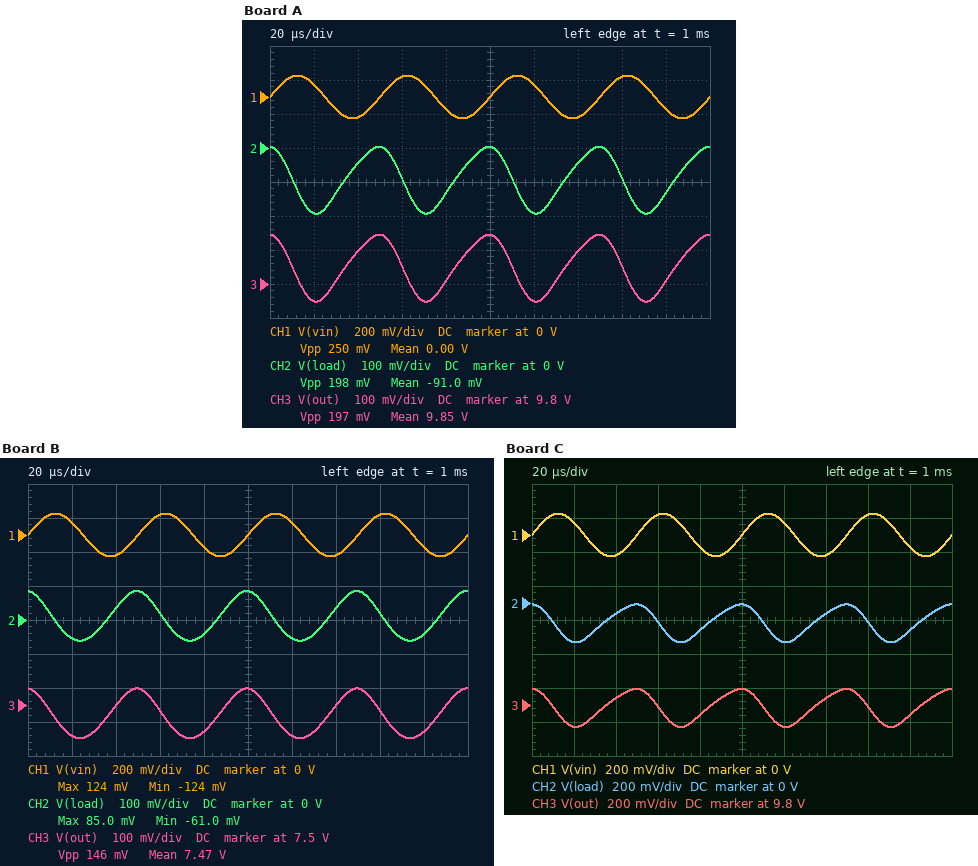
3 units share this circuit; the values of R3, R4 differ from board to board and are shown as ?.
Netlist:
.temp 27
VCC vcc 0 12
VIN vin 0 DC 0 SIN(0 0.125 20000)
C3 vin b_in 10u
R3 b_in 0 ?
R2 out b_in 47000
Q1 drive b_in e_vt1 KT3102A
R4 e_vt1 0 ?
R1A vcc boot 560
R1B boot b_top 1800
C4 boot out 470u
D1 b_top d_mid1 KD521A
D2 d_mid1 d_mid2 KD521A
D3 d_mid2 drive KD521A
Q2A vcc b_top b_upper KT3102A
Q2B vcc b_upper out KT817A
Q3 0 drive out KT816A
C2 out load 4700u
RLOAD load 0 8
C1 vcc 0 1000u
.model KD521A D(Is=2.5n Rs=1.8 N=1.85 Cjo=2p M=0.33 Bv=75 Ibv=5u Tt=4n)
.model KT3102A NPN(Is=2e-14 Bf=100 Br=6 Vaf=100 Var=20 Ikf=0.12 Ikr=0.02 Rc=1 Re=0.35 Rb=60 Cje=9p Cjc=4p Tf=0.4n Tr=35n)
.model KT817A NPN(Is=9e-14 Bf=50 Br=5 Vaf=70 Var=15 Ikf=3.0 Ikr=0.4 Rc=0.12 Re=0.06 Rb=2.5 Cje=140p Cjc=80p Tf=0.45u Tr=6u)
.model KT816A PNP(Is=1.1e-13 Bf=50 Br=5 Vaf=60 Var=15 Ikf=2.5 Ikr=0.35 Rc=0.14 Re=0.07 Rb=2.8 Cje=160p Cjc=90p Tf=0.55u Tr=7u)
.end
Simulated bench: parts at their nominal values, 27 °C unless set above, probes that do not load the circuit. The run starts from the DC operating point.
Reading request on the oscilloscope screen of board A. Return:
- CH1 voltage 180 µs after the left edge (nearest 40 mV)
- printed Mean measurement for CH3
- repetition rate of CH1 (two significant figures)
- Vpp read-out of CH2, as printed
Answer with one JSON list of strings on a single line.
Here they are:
["-80 mV", "9.85 V", "20 kHz", "198 mV"]
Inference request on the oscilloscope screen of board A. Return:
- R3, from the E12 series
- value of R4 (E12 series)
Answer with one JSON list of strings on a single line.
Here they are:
["3.3 kΩ", "68 Ω"]
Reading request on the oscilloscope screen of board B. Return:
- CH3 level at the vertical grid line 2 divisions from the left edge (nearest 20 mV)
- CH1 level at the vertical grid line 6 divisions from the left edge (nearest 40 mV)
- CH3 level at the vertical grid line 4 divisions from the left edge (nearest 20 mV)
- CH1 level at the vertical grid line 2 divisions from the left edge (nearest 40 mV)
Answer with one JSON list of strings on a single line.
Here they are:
["7.50 V", "80 mV", "7.42 V", "-120 mV"]
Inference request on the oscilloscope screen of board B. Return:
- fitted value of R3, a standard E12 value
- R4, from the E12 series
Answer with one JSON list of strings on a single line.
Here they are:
["8.2 kΩ", "220 Ω"]
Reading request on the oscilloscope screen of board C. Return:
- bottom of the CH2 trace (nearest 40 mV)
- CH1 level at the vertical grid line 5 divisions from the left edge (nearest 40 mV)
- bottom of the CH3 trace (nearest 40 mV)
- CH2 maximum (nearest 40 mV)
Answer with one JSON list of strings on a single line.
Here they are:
["-240 mV", "0 V", "9.68 V", "0 V"]
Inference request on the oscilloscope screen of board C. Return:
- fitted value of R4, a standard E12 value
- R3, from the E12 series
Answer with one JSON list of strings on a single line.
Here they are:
["56 Ω", "3.3 kΩ"]
